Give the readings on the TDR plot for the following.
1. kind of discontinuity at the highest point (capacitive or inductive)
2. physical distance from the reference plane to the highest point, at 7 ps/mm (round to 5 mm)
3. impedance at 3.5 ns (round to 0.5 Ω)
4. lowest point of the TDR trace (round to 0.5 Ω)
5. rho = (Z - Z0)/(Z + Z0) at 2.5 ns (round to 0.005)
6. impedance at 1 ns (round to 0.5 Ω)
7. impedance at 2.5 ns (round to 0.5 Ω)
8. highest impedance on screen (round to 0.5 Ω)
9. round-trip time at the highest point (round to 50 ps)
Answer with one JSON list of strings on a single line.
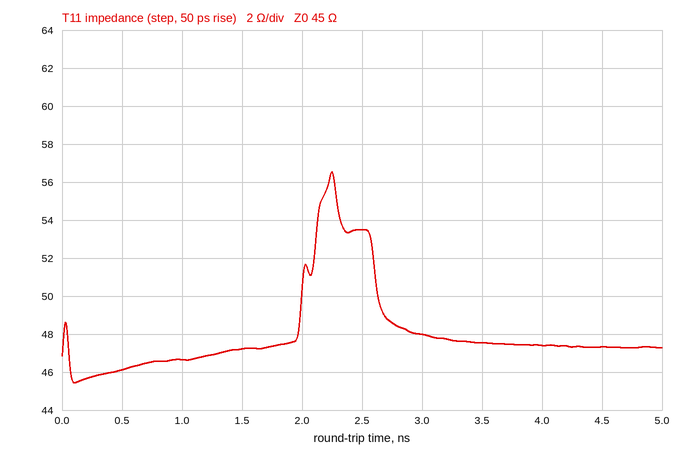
["inductive", "160 mm", "47.5 Ω", "45.5 Ω", "+0.085", "46.5 Ω", "53.5 Ω", "56.5 Ω", "2.25 ns"]
